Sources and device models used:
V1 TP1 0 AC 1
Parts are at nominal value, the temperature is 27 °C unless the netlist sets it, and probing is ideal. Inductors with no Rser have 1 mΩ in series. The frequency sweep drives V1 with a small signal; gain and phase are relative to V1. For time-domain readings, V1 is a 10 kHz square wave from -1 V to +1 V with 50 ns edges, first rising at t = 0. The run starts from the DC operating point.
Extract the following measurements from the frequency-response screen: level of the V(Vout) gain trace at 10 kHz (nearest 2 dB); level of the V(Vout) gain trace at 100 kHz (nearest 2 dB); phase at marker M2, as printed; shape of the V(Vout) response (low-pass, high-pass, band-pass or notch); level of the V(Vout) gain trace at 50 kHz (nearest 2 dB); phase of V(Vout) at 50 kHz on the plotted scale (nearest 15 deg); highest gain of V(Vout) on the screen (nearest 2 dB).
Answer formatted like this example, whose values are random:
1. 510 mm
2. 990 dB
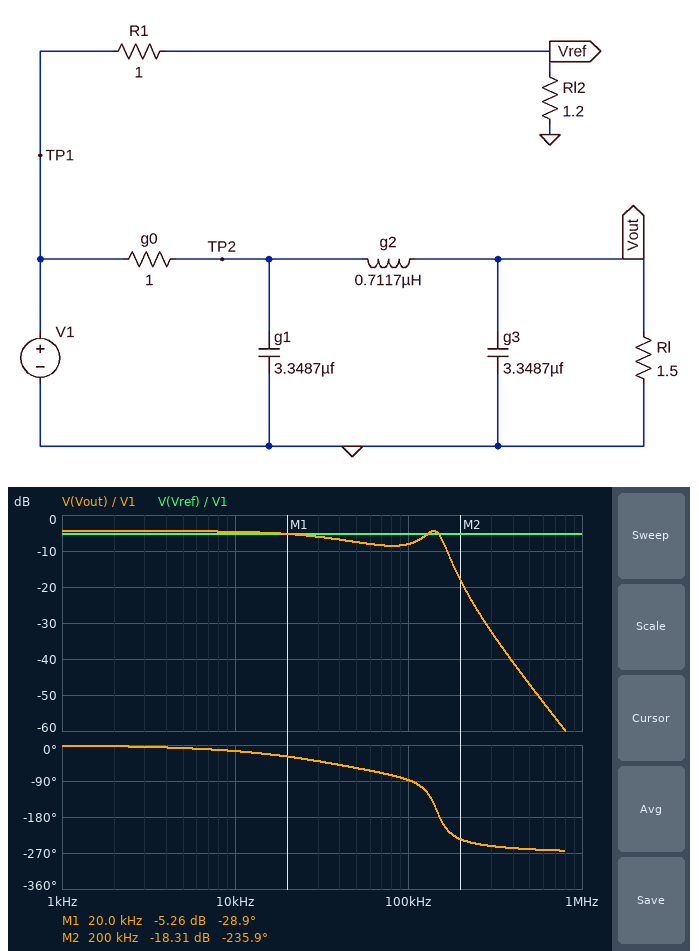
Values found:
1. -4 dB
2. -8 dB
3. -235.9 deg
4. low-pass
5. -8 dB
6. -60 deg
7. -4 dB
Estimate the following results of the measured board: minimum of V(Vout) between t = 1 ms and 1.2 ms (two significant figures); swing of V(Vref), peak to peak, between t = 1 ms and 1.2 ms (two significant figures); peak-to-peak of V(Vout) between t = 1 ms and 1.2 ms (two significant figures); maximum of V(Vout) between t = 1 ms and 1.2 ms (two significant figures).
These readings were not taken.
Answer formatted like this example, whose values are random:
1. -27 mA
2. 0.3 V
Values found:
1. -620 mV
2. 1.1 V
3. 1.2 V
4. 620 mV
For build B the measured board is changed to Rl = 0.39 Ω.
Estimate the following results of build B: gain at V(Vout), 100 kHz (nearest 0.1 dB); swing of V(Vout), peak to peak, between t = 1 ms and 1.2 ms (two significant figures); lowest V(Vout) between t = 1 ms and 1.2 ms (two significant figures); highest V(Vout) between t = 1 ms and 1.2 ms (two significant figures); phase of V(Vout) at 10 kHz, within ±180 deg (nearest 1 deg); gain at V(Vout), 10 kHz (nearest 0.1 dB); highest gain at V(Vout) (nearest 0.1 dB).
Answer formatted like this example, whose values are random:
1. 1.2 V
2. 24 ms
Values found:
1. -10.6 dB
2. 700 mV
3. -350 mV
4. 350 mV
5. -9 deg
6. -11.1 dB
7. -10.3 dB
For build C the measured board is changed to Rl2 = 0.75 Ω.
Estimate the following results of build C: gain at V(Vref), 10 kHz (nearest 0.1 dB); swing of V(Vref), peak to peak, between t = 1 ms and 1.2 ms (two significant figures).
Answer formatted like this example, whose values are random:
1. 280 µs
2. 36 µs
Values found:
1. -7.4 dB
2. 860 mV
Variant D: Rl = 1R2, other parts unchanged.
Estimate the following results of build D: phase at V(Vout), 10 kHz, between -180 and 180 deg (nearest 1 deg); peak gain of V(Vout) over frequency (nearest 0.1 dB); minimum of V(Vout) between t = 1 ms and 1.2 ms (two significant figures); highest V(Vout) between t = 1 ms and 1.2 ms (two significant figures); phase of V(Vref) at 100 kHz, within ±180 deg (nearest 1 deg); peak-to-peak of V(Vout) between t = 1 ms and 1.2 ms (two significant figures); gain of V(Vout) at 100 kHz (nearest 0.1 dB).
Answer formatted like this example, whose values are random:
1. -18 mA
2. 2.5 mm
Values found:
1. -14 deg
2. -5.3 dB
3. -570 mV
4. 570 mV
5. 0 deg
6. 1.1 V
7. -8.3 dB
